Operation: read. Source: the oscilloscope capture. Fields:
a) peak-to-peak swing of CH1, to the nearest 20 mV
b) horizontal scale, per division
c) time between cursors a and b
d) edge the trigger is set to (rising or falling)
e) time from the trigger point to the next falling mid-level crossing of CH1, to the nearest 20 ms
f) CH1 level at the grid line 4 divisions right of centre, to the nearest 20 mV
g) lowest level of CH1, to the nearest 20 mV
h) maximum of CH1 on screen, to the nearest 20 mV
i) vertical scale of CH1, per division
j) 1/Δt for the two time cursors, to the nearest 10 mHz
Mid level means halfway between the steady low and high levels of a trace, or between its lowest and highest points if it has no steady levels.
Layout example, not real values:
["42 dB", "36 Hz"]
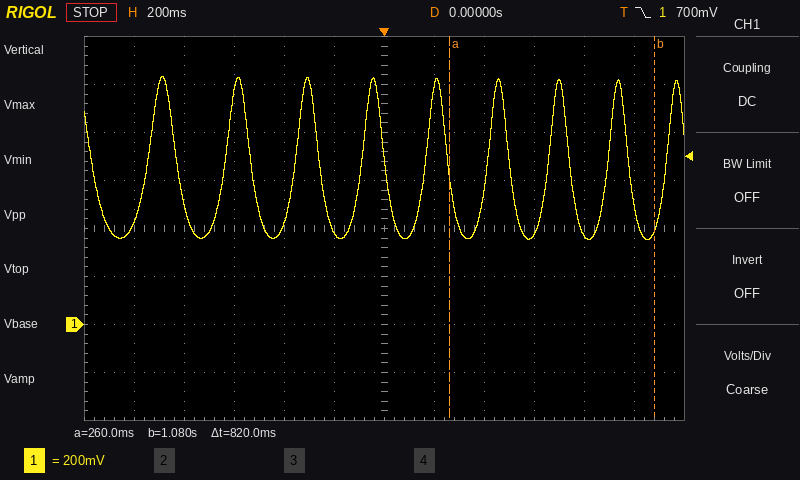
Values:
["680 mV", "200 ms", "820 ms", "falling", "260 ms", "380 mV", "360 mV", "1.04 V", "200 mV", "1.22 Hz"]
